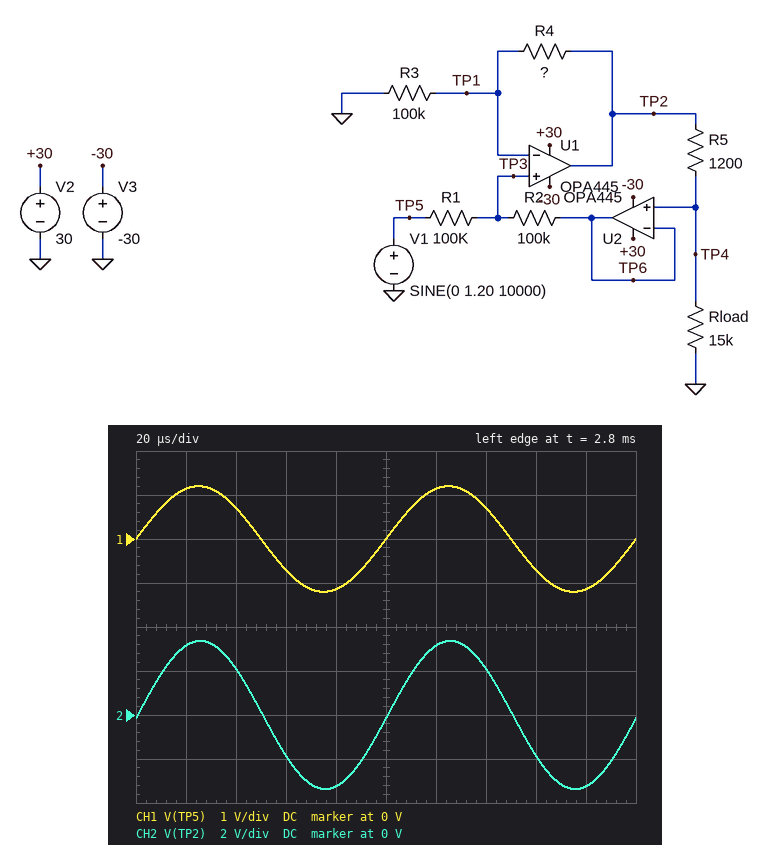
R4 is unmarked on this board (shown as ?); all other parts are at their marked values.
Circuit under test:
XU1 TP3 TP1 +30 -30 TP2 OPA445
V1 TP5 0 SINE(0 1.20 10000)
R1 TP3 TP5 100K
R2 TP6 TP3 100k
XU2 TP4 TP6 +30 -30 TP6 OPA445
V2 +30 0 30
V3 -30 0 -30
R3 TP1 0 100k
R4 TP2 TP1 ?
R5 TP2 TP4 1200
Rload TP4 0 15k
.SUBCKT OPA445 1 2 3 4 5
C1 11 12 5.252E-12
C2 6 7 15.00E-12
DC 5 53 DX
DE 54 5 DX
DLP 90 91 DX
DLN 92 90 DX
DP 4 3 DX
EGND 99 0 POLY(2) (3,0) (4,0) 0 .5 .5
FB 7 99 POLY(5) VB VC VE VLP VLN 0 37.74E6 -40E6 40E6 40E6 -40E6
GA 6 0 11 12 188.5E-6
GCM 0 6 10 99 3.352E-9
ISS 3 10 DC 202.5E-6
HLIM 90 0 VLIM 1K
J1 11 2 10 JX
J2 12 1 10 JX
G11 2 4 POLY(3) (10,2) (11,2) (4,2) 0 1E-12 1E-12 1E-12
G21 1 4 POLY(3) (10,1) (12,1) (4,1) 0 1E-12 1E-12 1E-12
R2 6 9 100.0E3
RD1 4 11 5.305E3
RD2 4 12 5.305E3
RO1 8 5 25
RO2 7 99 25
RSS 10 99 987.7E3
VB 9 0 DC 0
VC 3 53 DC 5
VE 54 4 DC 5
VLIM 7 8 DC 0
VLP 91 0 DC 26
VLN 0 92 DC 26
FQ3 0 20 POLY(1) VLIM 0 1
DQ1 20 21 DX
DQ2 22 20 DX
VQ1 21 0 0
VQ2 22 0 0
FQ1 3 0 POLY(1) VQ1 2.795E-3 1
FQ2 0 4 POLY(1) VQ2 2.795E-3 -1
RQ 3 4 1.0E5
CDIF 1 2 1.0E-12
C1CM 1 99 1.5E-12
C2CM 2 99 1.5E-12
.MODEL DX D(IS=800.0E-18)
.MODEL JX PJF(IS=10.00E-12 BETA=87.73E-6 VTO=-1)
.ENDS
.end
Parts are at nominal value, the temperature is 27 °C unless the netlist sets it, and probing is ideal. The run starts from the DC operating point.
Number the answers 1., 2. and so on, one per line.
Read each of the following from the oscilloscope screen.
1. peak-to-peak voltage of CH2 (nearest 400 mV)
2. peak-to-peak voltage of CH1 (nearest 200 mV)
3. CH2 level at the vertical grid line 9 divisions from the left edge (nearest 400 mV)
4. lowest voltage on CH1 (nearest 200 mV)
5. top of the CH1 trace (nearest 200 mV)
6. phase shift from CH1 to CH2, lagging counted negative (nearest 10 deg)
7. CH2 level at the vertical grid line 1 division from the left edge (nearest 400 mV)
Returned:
1. 6.8 V
2. 2.4 V
3. -3.2 V
4. -1.2 V
5. 1.2 V
6. 0 deg
7. 3.2 V
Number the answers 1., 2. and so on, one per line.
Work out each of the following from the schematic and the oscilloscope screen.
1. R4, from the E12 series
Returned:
1. 56 kΩ
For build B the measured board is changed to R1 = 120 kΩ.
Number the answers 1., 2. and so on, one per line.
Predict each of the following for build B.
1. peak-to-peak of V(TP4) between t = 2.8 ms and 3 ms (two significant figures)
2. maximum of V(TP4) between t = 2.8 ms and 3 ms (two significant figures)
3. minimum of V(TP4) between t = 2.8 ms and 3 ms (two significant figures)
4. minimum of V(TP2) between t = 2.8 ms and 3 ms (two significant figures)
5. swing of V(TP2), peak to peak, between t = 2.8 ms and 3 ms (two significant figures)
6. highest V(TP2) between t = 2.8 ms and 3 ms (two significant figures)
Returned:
1. 7.4 V
2. 3.7 V
3. -3.7 V
4. -4.0 V
5. 8.0 V
6. 4.0 V
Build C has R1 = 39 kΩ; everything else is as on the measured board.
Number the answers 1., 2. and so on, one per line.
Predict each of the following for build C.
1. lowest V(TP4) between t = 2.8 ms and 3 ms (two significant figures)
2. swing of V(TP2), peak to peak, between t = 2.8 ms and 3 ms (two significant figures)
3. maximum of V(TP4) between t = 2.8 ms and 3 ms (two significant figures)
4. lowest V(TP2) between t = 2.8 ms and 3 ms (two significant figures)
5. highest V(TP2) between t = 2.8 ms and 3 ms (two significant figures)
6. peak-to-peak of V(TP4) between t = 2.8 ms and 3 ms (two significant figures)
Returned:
1. -2.1 V
2. 4.5 V
3. 2.1 V
4. -2.3 V
5. 2.3 V
6. 4.2 V
